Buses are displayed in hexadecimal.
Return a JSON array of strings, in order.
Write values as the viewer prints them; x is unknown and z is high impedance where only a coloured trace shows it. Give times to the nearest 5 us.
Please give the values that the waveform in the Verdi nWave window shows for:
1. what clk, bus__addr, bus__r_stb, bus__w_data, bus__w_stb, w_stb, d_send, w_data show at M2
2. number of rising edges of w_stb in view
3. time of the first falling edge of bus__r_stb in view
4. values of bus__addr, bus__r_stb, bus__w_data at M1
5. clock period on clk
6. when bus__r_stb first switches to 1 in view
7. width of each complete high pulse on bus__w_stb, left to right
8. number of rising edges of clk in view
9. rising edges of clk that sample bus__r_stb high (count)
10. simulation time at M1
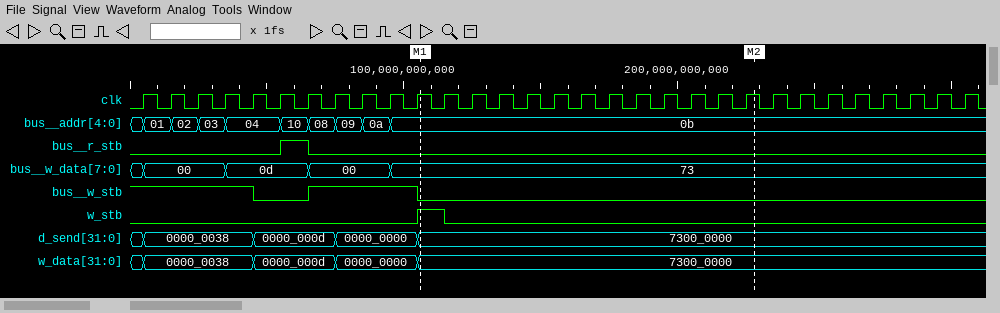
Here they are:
["clk=1, bus__addr=0b, bus__r_stb=0, bus__w_data=73, bus__w_stb=0, w_stb=0, d_send=7300_0000, w_data=7300_0000", "1", "65 us", "bus__addr=0b, bus__r_stb=0, bus__w_data=73", "10 us", "55 us", "40 us", "31", "1", "105 us"]
